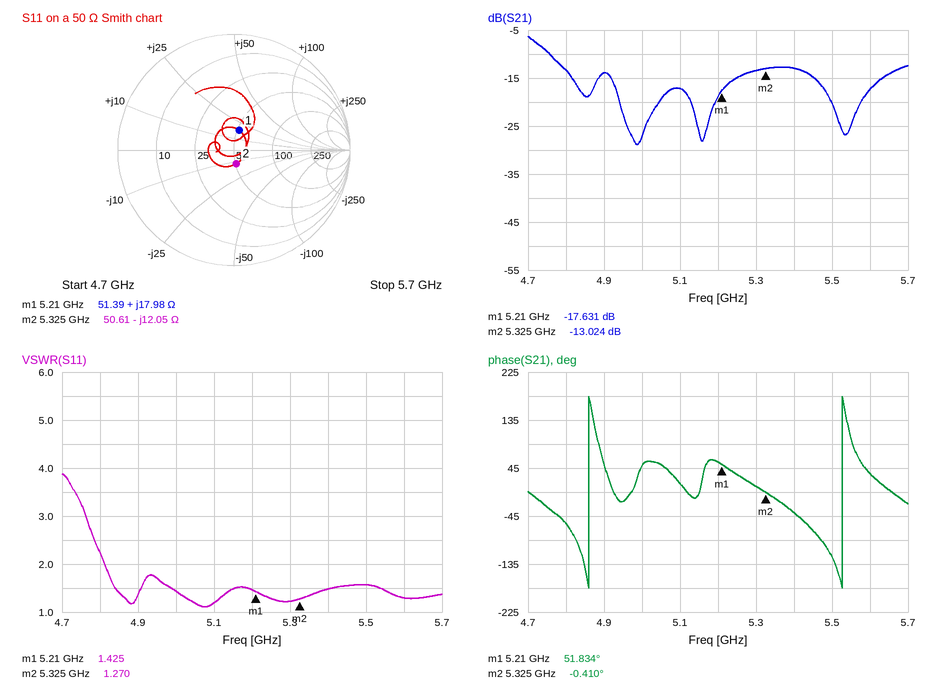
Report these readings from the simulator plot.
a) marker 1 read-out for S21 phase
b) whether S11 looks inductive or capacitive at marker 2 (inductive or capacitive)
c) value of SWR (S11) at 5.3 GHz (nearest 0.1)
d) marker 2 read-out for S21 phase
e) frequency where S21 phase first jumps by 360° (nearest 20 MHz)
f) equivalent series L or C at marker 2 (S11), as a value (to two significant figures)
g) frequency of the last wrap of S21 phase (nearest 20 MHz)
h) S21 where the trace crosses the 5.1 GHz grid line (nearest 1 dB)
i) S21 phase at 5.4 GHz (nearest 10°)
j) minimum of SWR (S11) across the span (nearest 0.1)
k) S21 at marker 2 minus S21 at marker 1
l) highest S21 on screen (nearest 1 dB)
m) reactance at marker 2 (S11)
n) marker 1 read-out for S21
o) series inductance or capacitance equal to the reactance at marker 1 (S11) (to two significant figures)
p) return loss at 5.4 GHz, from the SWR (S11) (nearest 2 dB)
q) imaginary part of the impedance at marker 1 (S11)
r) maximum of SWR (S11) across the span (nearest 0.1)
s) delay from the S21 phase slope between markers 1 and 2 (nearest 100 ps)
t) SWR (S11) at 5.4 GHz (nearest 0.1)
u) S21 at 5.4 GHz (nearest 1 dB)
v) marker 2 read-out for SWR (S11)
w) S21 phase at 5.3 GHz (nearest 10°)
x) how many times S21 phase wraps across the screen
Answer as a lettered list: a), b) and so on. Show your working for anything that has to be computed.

a) 51.834°
b) capacitive
c) 1.2
d) -0.410°
e) 4.86 GHz
f) C = 1/(2π × 5.325 GHz × 12.05 Ω) ≈ 2.5 pF
g) 5.52 GHz
h) -17 dB
i) -40°
j) 1.1
k) -13.024 − (-17.631) = 4.607 dB
l) -6 dB
m) -12.05 Ω
n) -17.631 dB
o) L = 17.98 Ω/(2π × 5.21 GHz) ≈ 549 pH, so 550 pH to two significant figures
p) −20 log10((1.5 − 1)/(1.5 + 1)) ≈ 14 dB
q) +17.98 Ω
r) 3.9
s) −(-0.41° − (51.834°))/(360° × 115 MHz) ≈ 1.3 ns
t) 1.5
u) -13 dB
v) 1.270
w) 10°
x) 2
